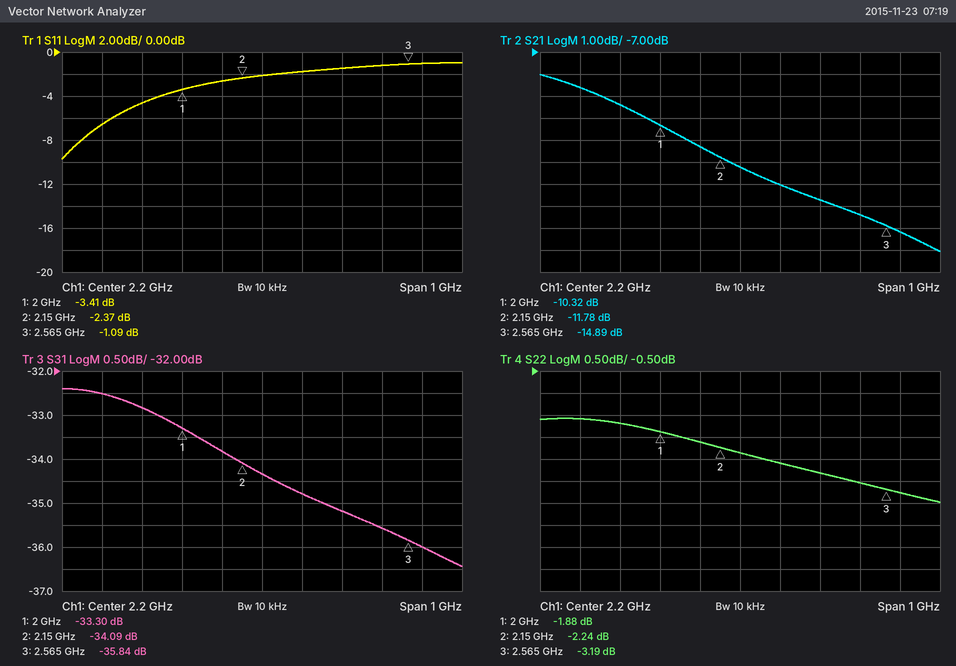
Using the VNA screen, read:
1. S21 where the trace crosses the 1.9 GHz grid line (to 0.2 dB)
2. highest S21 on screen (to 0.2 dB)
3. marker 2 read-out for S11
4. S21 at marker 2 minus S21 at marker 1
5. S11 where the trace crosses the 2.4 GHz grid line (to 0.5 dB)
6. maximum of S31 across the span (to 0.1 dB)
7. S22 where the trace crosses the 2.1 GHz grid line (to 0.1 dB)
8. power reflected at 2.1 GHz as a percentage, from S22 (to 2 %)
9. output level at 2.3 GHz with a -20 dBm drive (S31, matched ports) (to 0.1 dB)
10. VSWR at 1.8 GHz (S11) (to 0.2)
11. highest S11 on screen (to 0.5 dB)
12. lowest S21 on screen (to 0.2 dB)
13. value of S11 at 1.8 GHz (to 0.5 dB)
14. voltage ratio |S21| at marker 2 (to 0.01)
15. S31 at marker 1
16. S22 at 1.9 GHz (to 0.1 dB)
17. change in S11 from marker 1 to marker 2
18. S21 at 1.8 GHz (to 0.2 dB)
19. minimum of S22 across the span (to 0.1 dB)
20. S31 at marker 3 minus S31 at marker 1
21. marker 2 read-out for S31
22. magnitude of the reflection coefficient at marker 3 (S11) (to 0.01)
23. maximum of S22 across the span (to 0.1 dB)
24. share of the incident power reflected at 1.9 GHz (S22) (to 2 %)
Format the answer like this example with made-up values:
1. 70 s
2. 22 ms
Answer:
1. -9.4 dB
2. -8.0 dB
3. -2.37 dB
4. -1.46 dB
5. -1.5 dB
6. -32.4 dB
7. -2.1 dB
8. 62 %
9. -54.8 dBm
10. 2.8
11. -1.0 dB
12. -16.0 dB
13. -6.5 dB
14. 0.26
15. -33.30 dB
16. -1.7 dB
17. 1.04 dB
18. -8.6 dB
19. -3.5 dB
20. -2.54 dB
21. -34.09 dB
22. 0.88
23. -1.6 dB
24. 68 %
